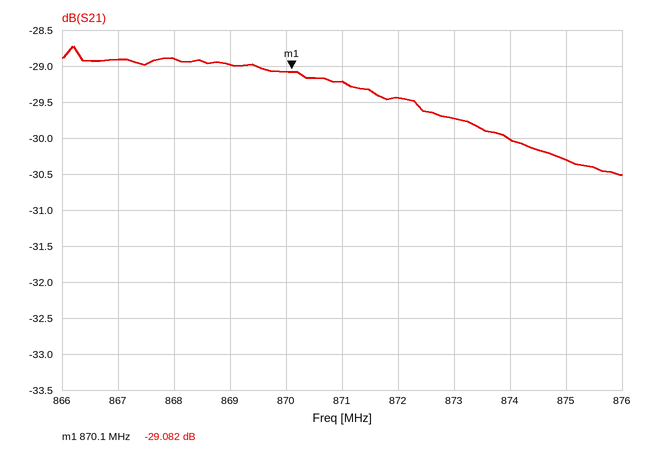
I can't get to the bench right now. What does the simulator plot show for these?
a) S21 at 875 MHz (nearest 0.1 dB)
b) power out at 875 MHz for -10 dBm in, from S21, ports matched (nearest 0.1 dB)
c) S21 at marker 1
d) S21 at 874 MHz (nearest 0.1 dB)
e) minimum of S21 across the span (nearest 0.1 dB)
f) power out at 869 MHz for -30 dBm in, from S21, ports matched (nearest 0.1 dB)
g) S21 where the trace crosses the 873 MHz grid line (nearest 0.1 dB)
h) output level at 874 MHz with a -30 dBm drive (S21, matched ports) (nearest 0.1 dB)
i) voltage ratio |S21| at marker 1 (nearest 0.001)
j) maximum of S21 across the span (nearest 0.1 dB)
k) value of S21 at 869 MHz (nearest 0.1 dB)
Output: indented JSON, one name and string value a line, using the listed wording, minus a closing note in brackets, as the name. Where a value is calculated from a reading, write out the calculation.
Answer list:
{
  "S21 at 875 MHz": "-30.3 dB",
  "power out at 875 MHz for -10 dBm in, from S21, ports matched": "-10 dBm + (-30.3 dB) = -40.3 dBm",
  "S21 at marker 1": "-29.082 dB",
  "S21 at 874 MHz": "-30.0 dB",
  "minimum of S21 across the span": "-30.5 dB",
  "power out at 869 MHz for -30 dBm in, from S21, ports matched": "-30 dBm + (-29.0 dB) = -59.0 dBm",
  "S21 where the trace crosses the 873 MHz grid line": "-29.7 dB",
  "output level at 874 MHz with a -30 dBm drive (S21, matched ports)": "-30 dBm + (-30.0 dB) = -60.0 dBm",
  "voltage ratio |S21| at marker 1": "10^(-29.082/20) ≈ 0.035",
  "maximum of S21 across the span": "-28.7 dB",
  "value of S21 at 869 MHz": "-29.0 dB"
}
